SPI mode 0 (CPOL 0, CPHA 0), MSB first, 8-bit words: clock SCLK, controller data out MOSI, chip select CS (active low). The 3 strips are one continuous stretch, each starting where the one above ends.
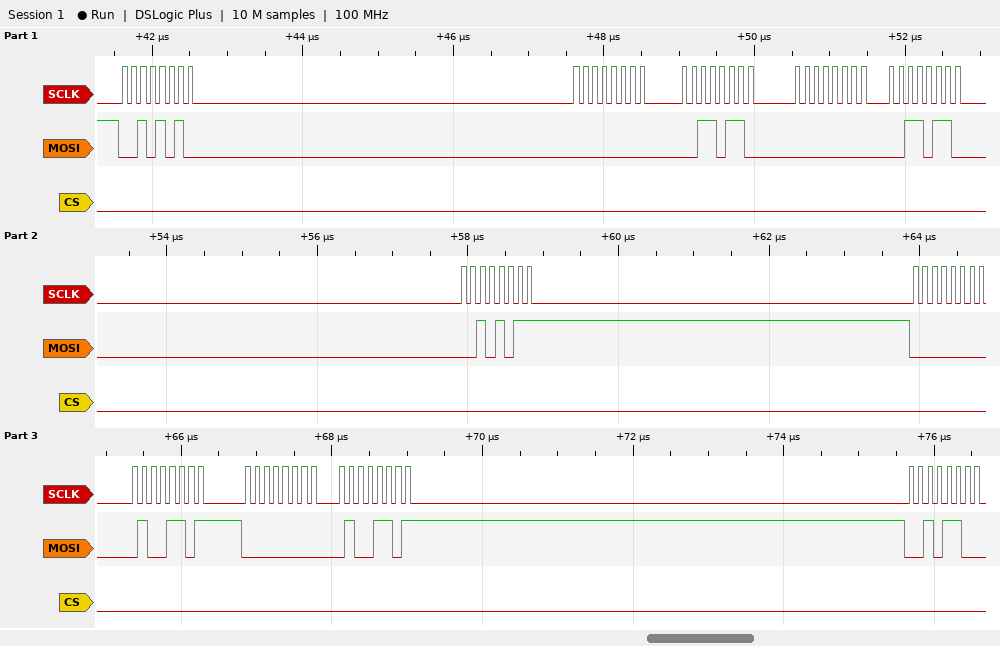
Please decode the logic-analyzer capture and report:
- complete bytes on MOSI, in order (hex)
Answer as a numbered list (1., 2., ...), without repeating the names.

1. 0x2A 0x00 0x36 0x00 0x36 0x2B 0x00 0x4D 0x00 0x4D 0x2C
